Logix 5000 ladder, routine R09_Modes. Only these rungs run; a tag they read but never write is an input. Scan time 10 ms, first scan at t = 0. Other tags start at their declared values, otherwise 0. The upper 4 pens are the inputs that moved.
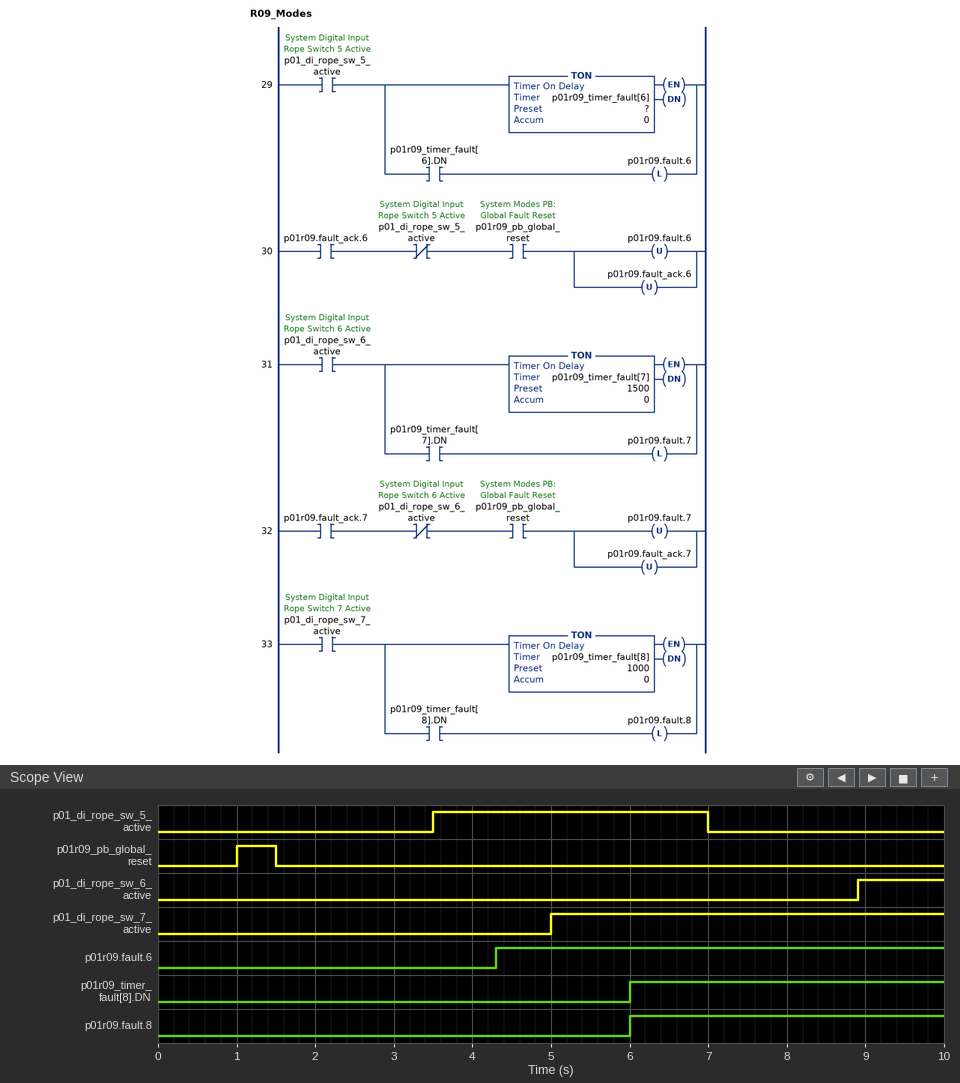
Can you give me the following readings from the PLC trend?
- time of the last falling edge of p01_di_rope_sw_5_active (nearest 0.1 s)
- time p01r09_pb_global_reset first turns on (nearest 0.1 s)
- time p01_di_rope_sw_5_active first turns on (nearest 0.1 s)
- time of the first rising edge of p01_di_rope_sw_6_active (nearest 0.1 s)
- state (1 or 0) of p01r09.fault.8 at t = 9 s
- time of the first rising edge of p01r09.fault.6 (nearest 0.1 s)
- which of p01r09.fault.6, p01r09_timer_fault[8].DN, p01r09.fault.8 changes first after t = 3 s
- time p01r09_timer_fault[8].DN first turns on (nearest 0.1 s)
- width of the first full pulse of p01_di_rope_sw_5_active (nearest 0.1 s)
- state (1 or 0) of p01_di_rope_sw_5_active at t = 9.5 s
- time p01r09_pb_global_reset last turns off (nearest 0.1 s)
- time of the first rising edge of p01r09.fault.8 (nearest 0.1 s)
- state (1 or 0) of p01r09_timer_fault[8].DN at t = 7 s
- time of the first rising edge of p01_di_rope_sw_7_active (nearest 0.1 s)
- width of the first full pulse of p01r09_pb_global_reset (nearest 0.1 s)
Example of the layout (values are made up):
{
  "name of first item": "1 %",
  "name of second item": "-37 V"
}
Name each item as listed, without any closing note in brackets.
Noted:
{
  "time of the last falling edge of p01_di_rope_sw_5_active": "7.0 s",
  "time p01r09_pb_global_reset first turns on": "1.0 s",
  "time p01_di_rope_sw_5_active first turns on": "3.5 s",
  "time of the first rising edge of p01_di_rope_sw_6_active": "8.9 s",
  "state (1 or 0) of p01r09.fault.8 at t = 9 s": "1",
  "time of the first rising edge of p01r09.fault.6": "4.3 s",
  "which of p01r09.fault.6, p01r09_timer_fault[8].DN, p01r09.fault.8 changes first after t = 3 s": "p01r09.fault.6",
  "time p01r09_timer_fault[8].DN first turns on": "6.0 s",
  "width of the first full pulse of p01_di_rope_sw_5_active": "3.5 s",
  "state (1 or 0) of p01_di_rope_sw_5_active at t = 9.5 s": "0",
  "time p01r09_pb_global_reset last turns off": "1.5 s",
  "time of the first rising edge of p01r09.fault.8": "6.0 s",
  "state (1 or 0) of p01r09_timer_fault[8].DN at t = 7 s": "1",
  "time of the first rising edge of p01_di_rope_sw_7_active": "5.0 s",
  "width of the first full pulse of p01r09_pb_global_reset": "0.5 s"
}
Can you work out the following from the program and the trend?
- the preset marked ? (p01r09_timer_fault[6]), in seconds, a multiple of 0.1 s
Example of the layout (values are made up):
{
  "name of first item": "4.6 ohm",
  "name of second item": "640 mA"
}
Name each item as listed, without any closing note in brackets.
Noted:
{
  "the preset marked ? (p01r09_timer_fault[6]), in seconds, a multiple of 0.1 s": "0.8 s"
}
